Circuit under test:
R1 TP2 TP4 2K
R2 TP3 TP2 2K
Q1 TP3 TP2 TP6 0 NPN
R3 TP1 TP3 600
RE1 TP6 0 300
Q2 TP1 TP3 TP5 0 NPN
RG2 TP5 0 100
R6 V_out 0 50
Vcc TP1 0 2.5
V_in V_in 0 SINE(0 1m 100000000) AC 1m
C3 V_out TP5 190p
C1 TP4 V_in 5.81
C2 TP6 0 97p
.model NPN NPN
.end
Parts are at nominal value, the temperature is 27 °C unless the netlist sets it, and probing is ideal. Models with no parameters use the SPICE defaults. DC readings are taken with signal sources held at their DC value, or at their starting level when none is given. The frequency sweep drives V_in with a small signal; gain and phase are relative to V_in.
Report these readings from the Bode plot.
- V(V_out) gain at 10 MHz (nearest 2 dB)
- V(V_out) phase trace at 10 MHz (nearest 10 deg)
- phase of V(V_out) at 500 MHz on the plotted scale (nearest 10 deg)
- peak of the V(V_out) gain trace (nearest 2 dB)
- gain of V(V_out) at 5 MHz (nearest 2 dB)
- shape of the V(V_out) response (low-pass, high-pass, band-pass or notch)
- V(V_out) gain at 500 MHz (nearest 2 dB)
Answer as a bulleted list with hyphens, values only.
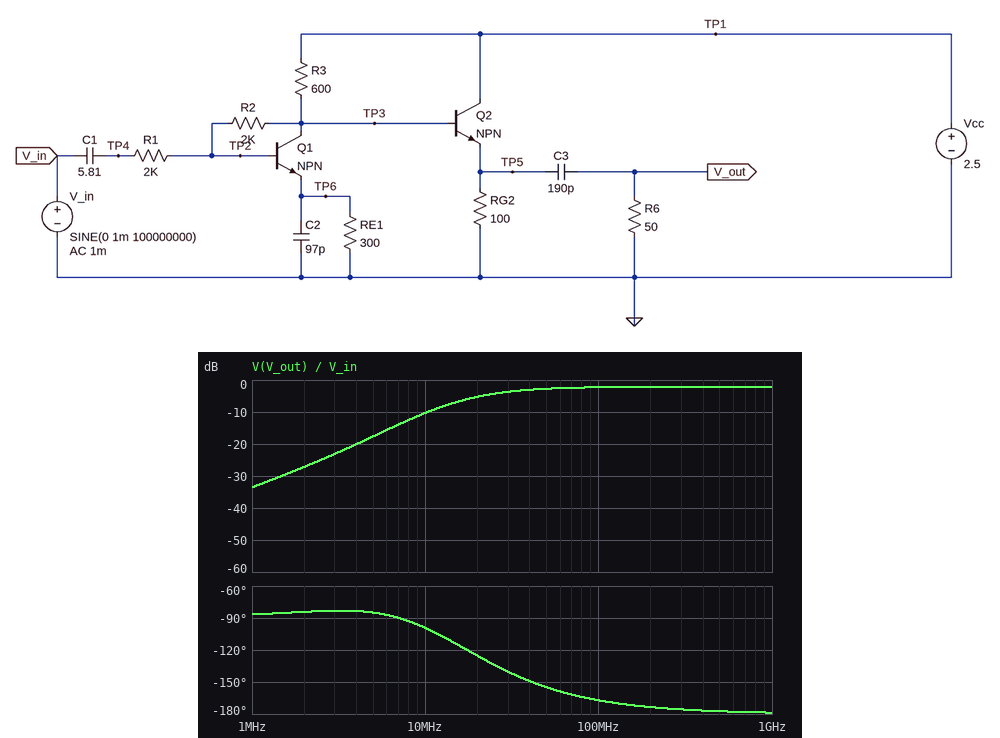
- -10 dB
- -100 deg
- -180 deg
- -2 dB
- -18 dB
- high-pass
- -2 dB
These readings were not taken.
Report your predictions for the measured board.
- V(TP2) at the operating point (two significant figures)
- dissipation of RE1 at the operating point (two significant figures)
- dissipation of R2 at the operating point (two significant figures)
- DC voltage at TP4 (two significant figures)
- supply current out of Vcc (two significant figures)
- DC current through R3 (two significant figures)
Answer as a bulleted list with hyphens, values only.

- 1.3 V
- 1.0 mW
- 650 nW
- 1.3 V
- 7.4 mA
- 1.9 mA
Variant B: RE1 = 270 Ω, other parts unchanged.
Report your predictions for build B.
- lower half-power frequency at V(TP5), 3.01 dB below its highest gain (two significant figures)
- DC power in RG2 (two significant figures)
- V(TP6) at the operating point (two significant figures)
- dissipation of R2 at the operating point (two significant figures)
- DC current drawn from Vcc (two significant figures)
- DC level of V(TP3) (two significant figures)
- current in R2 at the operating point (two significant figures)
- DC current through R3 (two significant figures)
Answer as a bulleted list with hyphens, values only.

- 8.1 MHz
- 2.7 mW
- 510 mV
- 700 nW
- 7.1 mA
- 1.3 V
- 19 µA
- 1.9 mA
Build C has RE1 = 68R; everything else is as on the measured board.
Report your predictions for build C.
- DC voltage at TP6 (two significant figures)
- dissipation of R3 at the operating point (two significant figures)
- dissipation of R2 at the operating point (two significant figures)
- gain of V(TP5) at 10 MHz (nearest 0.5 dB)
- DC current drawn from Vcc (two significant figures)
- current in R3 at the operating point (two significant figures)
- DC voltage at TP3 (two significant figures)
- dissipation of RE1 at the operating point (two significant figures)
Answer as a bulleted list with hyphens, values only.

- 170 mV
- 3.7 mW
- 1.2 µW
- -4.5 dB
- 4.6 mA
- 2.5 mA
- 1.0 V
- 410 µW
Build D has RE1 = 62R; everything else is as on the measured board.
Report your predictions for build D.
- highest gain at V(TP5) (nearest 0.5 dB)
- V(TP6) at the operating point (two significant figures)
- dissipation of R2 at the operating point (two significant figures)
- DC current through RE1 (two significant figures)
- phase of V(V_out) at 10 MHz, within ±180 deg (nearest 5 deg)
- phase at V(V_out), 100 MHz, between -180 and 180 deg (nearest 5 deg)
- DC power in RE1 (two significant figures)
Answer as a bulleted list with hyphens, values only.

- -3.5 dB
- 150 mV
- 1.2 µW
- 2.5 mA
- -120 deg
- -170 deg
- 380 µW
